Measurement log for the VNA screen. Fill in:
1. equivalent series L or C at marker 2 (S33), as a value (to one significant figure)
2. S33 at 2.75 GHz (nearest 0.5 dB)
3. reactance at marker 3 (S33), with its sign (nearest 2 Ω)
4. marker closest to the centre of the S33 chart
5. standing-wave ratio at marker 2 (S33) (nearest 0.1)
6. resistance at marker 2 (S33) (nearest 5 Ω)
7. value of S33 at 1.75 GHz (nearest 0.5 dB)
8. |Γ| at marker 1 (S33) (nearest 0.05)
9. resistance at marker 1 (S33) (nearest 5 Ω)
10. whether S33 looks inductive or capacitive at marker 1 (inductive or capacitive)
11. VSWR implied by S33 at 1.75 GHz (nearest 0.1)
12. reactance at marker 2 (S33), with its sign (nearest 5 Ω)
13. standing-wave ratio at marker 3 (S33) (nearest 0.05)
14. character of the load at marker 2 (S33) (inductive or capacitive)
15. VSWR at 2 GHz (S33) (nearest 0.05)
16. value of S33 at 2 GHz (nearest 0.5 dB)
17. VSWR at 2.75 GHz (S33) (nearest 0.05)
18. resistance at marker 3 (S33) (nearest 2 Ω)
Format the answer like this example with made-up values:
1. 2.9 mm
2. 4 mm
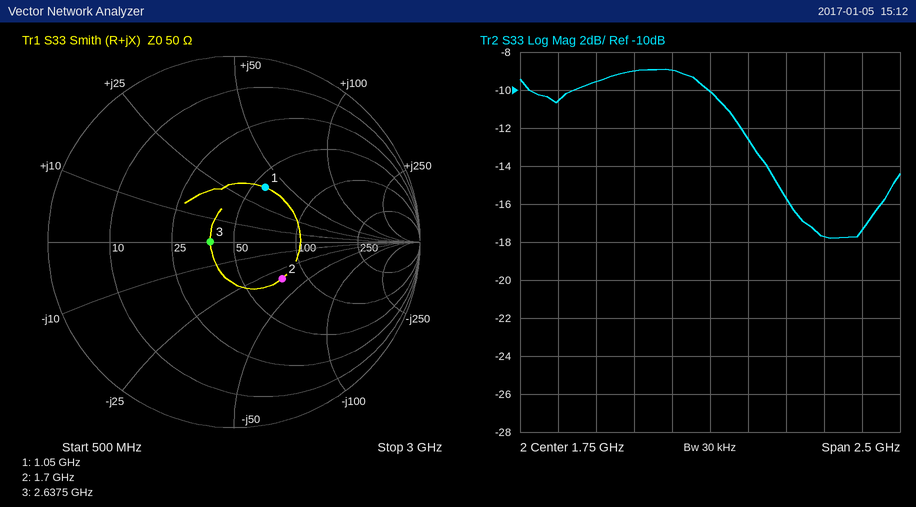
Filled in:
1. 3 pF
2. -17.5 dB
3. 0 Ω
4. marker 3
5. 2.0
6. 75 Ω
7. -10.0 dB
8. 0.35
9. 55 Ω
10. inductive
11. 1.9
12. -35 Ω
13. 1.30
14. capacitive
15. 1.60
16. -12.5 dB
17. 1.30
18. 38 Ω
